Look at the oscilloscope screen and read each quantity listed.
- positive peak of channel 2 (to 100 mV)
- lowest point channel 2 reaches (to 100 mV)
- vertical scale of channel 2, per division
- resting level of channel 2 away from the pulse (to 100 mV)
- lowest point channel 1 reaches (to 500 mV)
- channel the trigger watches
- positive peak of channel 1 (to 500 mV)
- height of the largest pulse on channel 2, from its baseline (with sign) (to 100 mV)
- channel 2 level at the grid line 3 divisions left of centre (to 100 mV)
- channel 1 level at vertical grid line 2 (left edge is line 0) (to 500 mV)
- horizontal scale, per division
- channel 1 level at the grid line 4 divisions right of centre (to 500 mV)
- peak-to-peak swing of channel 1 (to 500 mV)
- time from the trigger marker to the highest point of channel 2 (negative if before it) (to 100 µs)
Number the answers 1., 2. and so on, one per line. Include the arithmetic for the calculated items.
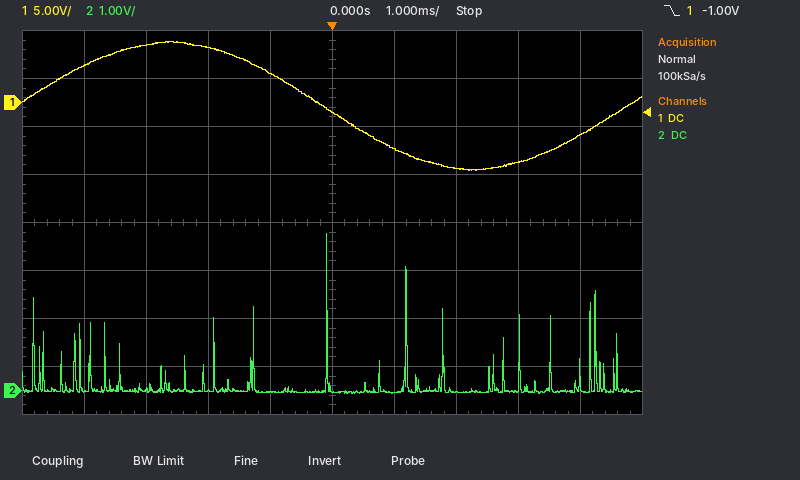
1. 3.3 V
2. -100 mV
3. 1 V
4. 0.0 V
5. -7.0 V
6. channel 1
7. 6.5 V
8. 3.3 V − (0.0 V) = +3.3 V
9. 0.0 V
10. 6.0 V
11. 1 ms
12. -3.5 V
13. 6.5 V − (-7.0 V) = 13.5 V
14. -100 µs
